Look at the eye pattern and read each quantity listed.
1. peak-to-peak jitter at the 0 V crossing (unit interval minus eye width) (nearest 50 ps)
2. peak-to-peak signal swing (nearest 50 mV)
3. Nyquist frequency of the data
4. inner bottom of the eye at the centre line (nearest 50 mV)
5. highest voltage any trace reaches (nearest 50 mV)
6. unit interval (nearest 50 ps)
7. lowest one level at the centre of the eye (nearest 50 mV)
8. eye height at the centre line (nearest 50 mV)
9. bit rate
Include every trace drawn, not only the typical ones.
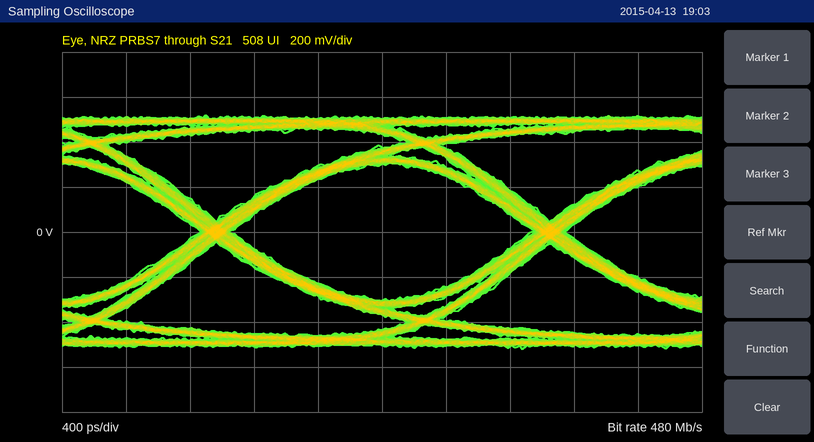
200 ps
1.05 V
240 MHz
-300 mV
500 mV
2.10 ns
300 mV
600 mV
480 Mb/s
